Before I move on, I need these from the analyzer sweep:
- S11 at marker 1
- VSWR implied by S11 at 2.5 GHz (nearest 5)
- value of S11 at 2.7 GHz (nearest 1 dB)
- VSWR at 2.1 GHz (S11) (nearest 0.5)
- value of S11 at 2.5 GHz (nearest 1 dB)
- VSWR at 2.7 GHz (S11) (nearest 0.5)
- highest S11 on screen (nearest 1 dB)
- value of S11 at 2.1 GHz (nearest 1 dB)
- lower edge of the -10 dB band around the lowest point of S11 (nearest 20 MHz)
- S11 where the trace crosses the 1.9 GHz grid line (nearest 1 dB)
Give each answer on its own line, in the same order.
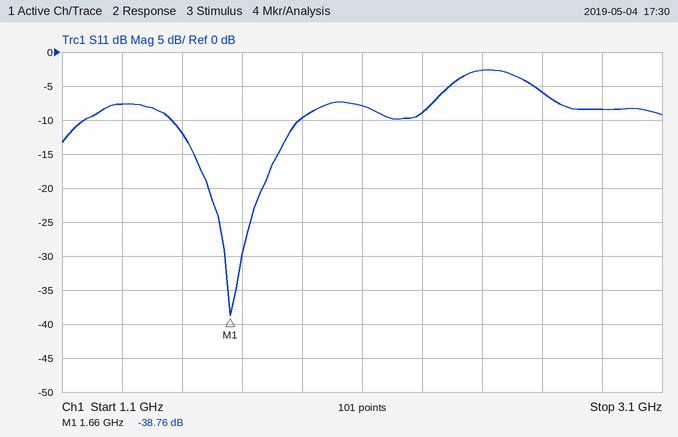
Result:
-38.76 dB
5
-6 dB
2.5
-3 dB
3.0
-3 dB
-8 dB
1.46 GHz
-10 dB
